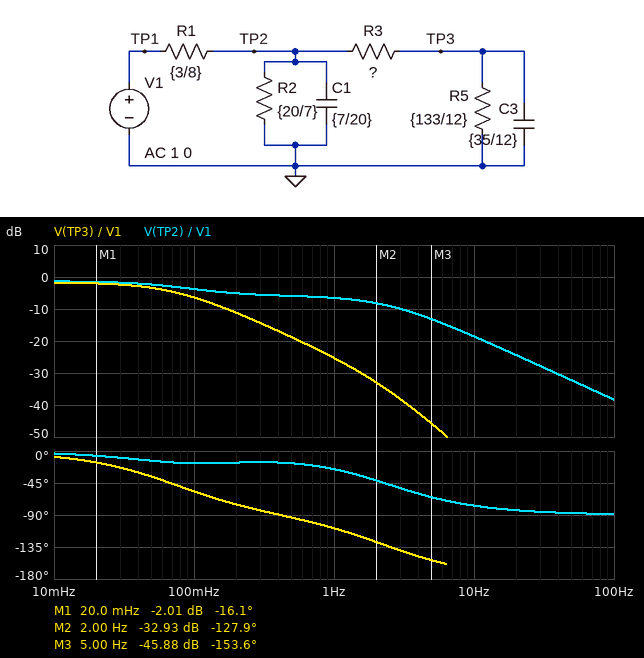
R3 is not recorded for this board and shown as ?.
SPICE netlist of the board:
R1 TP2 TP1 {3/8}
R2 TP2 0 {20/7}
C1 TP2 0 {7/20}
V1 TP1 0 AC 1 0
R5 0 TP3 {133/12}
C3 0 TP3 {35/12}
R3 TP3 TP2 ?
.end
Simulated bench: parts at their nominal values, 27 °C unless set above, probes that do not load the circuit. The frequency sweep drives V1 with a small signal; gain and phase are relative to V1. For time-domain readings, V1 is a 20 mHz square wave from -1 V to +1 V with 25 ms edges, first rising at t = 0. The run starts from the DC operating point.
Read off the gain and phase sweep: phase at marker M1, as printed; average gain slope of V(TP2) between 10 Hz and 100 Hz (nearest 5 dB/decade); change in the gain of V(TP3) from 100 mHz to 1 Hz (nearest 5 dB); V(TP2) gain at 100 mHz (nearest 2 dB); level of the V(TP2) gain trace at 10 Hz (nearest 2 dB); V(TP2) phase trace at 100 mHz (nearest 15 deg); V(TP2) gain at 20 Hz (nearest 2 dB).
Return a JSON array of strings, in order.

["-16.1 deg", "-20 dB/decade", "-20 dB", "-4 dB", "-18 dB", "-15 deg", "-24 dB"]
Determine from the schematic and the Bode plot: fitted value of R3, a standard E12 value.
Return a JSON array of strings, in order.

["0.47 Ω"]
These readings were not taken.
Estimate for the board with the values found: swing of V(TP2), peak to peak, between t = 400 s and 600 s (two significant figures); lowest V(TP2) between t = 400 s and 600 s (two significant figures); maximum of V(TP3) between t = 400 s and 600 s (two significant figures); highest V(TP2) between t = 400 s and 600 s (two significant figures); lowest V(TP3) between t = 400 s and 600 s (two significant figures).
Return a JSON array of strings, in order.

["1.7 V", "-860 mV", "820 mV", "860 mV", "-820 mV"]
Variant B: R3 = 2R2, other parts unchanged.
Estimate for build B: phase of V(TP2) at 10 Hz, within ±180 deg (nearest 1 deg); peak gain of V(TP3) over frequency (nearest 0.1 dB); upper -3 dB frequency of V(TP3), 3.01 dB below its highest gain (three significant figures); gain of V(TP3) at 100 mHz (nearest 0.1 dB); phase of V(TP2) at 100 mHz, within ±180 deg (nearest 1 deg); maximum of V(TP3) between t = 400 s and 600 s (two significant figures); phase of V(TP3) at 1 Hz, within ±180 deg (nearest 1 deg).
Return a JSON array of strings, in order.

["-81 deg", "-2.9 dB", "26.4 mHz", "-14.7 dB", "-5 deg", "700 mV", "-121 deg"]
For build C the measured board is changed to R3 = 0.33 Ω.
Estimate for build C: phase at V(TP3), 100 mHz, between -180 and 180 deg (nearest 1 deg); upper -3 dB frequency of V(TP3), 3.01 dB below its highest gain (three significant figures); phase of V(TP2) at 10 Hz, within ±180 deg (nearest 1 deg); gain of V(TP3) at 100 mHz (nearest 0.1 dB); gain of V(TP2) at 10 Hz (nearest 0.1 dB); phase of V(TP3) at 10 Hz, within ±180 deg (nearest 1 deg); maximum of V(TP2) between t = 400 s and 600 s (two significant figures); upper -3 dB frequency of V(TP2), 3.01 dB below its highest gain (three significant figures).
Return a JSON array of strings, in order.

["-52 deg", "84.7 mHz", "-75 deg", "-5.4 dB", "-18.7 dB", "-164 deg", "860 mV", "119 mHz"]
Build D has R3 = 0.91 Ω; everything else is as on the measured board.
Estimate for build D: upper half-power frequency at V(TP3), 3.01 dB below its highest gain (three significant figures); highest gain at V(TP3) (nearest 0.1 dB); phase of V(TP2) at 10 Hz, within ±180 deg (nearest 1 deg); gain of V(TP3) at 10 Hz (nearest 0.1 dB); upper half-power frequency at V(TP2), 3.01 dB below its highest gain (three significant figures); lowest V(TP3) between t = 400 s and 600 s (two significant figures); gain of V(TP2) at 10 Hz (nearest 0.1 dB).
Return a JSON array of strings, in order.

["48.4 mHz", "-2.0 dB", "-79 deg", "-62.9 dB", "654 mHz", "-790 mV", "-18.5 dB"]
